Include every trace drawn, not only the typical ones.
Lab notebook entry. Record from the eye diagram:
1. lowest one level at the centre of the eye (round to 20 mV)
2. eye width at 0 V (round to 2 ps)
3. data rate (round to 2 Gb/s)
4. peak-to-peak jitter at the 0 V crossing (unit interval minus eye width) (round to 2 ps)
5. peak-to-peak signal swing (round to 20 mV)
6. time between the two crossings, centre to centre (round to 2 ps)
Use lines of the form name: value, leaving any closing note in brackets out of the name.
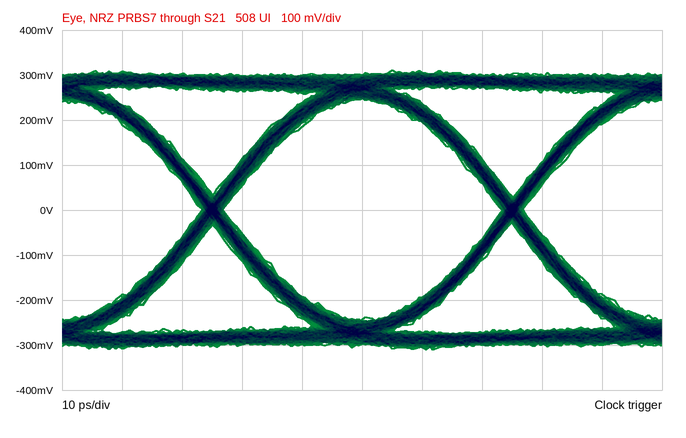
lowest one level at the centre of the eye: 240 mV
eye width at 0 V: 46 ps
data rate: 20 Gb/s
peak-to-peak jitter at the 0 V crossing (unit interval minus eye width): 4 ps
peak-to-peak signal swing: 620 mV
time between the two crossings, centre to centre: 50 ps
